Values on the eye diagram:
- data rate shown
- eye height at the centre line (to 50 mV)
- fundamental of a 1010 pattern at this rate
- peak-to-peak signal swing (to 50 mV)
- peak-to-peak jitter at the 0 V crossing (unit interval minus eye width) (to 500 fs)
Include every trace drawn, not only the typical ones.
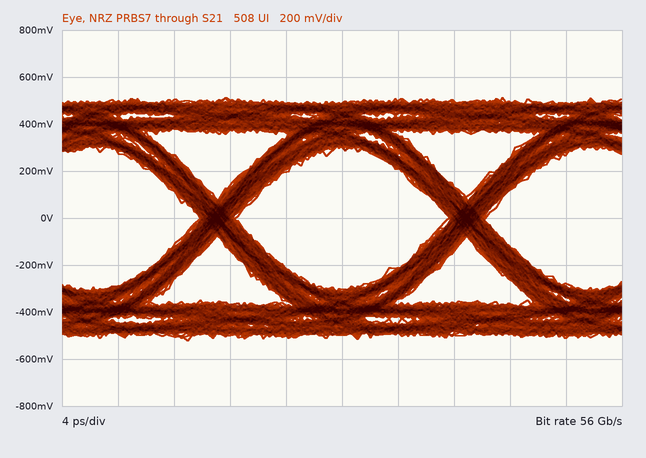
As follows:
56 Gb/s
600 mV
28 GHz
1.05 V
2.5 ps
